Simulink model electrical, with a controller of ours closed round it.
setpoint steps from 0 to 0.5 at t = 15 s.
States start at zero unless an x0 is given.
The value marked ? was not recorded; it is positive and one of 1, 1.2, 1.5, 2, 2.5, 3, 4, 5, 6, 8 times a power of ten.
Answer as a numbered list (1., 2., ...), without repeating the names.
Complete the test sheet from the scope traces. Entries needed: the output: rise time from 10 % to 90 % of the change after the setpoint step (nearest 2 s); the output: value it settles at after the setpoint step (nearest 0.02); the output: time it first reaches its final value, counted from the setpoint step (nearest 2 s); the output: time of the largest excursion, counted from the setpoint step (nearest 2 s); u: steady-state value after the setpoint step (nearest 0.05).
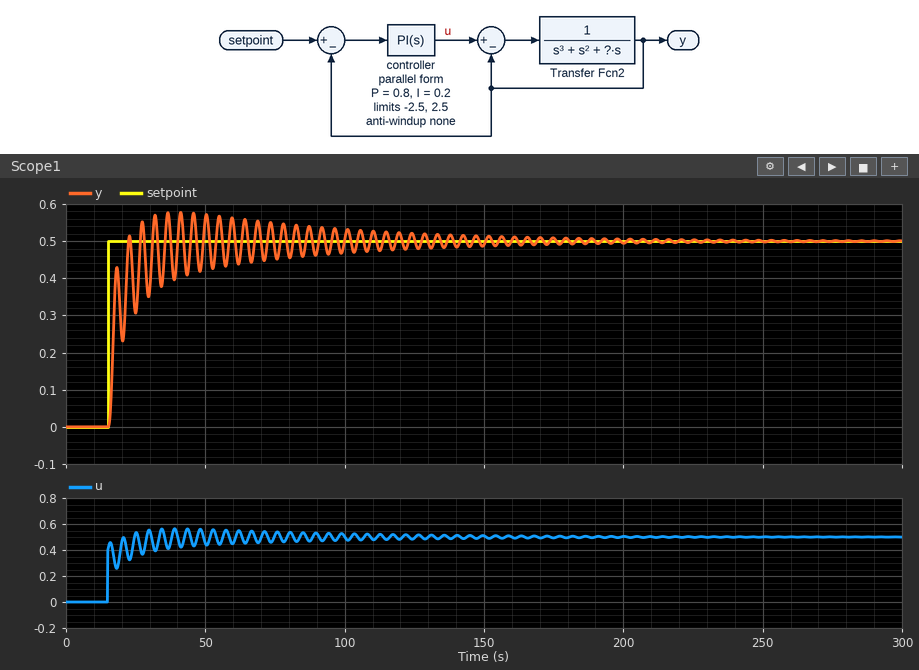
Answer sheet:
1. 6 s
2. 0.50
3. 8 s
4. 26 s
5. 0.50
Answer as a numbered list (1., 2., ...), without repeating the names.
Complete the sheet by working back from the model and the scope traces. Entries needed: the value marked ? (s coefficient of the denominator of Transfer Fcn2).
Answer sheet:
1. 2
